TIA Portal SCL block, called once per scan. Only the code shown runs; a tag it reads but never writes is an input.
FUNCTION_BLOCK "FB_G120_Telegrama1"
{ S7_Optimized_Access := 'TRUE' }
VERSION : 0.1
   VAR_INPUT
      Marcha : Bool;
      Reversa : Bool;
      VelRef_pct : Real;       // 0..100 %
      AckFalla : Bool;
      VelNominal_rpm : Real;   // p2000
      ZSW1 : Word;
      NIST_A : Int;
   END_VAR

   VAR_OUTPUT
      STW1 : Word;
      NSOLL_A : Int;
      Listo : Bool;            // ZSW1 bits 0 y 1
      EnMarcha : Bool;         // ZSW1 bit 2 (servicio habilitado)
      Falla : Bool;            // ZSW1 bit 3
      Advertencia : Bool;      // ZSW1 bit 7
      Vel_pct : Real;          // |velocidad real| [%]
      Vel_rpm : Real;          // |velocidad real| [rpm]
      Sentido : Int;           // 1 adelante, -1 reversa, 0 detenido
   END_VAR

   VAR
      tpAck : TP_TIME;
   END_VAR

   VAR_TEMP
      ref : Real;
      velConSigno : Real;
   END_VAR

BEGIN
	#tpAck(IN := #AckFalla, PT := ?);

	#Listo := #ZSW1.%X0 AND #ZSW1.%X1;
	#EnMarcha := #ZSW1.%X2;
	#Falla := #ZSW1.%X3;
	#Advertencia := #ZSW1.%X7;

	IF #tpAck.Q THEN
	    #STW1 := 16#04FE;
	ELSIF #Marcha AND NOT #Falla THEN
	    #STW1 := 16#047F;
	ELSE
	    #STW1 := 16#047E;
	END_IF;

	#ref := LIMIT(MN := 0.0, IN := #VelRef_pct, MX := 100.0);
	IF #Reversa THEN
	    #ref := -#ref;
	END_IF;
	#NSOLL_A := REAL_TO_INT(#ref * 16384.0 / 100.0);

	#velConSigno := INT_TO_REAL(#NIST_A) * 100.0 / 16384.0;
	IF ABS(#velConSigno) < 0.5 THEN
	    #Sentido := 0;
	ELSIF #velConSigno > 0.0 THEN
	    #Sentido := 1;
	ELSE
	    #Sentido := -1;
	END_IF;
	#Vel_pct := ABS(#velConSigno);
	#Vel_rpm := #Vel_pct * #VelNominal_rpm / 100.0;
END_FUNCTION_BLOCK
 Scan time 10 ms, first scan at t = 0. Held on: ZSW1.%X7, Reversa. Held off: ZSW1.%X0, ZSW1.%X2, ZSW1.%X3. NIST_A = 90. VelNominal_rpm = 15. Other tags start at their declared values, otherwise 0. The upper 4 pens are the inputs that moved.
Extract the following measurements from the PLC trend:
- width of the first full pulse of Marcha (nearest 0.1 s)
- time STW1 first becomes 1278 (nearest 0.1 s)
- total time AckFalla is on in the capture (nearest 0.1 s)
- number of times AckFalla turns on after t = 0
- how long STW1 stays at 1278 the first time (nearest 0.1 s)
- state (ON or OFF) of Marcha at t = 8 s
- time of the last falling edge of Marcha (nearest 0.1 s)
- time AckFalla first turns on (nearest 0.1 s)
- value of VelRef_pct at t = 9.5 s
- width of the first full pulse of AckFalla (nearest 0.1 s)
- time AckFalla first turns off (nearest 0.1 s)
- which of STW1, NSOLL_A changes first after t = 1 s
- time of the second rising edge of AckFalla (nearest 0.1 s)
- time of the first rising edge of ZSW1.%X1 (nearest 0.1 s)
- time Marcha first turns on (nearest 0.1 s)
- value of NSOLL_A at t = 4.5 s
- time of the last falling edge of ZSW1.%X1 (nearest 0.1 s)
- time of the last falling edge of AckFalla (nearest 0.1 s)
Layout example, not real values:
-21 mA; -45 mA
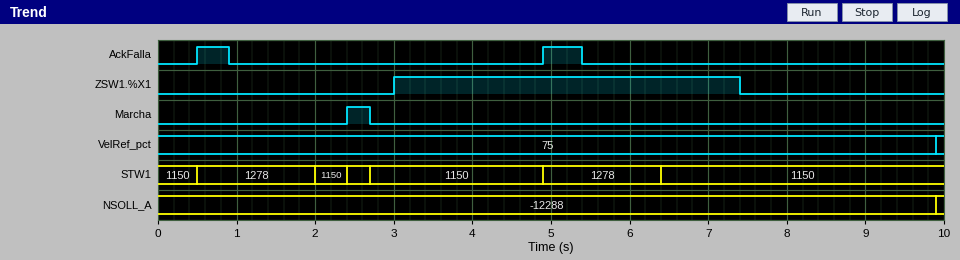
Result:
0.3 s; 0.5 s; 0.9 s; 2; 1.5 s; OFF; 2.7 s; 0.5 s; 75; 0.4 s; 0.9 s; STW1; 4.9 s; 3.0 s; 2.4 s; -12288; 7.4 s; 5.4 s
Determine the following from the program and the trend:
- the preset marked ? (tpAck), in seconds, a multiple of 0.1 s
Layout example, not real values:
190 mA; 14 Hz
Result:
1.5 s
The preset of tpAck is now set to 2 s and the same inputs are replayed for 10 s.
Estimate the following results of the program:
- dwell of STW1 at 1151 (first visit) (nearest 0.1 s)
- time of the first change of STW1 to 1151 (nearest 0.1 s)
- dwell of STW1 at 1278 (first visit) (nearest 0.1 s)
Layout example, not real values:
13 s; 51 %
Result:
0.2 s; 2.5 s; 2.0 s
